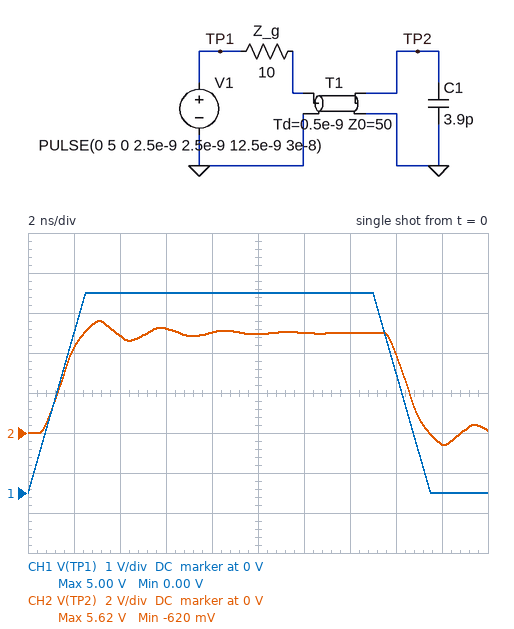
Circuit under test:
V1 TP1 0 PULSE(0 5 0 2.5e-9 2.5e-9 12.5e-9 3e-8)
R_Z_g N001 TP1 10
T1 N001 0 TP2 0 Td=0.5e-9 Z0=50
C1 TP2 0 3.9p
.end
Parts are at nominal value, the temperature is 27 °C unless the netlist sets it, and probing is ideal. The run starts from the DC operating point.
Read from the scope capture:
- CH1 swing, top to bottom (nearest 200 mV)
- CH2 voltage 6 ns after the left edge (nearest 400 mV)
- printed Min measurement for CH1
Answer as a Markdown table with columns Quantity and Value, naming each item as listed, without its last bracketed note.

| Quantity | Value |
|---|---|
| CH1 swing, top to bottom | 5.0 V |
| CH2 voltage 6 ns after the left edge | 5.2 V |
| printed Min measurement for CH1 | 0.00 V |
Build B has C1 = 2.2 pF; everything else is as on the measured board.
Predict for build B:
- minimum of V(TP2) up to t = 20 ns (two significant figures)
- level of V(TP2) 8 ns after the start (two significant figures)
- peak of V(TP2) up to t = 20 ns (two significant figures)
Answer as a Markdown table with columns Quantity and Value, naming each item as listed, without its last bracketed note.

| Quantity | Value |
|---|---|
| minimum of V(TP2) up to t = 20 ns | -500 mV |
| level of V(TP2) 8 ns after the start | 5.1 V |
| peak of V(TP2) up to t = 20 ns | 5.5 V |
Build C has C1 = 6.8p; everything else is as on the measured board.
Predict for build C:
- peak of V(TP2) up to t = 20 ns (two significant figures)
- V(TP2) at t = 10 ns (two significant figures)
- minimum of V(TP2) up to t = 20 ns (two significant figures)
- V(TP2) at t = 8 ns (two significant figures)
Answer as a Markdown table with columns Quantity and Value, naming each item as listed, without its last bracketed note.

| Quantity | Value |
|---|---|
| peak of V(TP2) up to t = 20 ns | 6.1 V |
| V(TP2) at t = 10 ns | 5.1 V |
| minimum of V(TP2) up to t = 20 ns | -1.1 V |
| V(TP2) at t = 8 ns | 4.7 V |
